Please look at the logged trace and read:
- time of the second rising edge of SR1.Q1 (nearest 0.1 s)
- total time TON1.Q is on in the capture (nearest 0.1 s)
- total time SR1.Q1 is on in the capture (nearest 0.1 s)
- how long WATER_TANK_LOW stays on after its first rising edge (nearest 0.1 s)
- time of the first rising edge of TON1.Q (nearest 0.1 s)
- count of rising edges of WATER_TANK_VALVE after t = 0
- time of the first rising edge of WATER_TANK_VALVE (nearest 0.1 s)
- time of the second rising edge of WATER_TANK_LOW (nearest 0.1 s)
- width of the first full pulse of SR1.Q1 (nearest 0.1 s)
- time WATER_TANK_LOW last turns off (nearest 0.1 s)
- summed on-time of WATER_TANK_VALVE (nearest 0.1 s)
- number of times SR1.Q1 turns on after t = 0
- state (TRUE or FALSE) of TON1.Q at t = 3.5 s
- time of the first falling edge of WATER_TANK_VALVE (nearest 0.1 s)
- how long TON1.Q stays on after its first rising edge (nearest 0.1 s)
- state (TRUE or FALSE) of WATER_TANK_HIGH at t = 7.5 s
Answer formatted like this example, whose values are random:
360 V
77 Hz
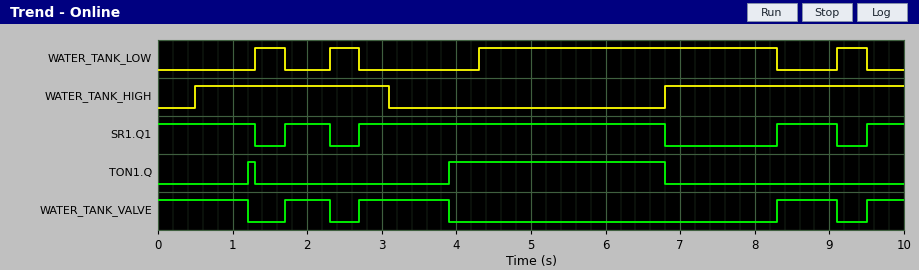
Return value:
2.7 s
3.0 s
7.3 s
0.4 s
1.2 s
4
1.7 s
2.3 s
0.6 s
9.5 s
4.3 s
4
FALSE
1.2 s
0.1 s
TRUE
